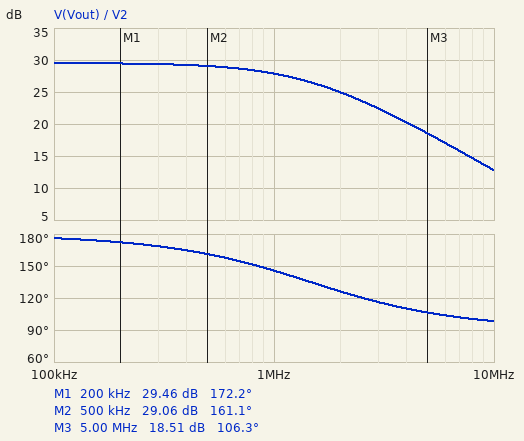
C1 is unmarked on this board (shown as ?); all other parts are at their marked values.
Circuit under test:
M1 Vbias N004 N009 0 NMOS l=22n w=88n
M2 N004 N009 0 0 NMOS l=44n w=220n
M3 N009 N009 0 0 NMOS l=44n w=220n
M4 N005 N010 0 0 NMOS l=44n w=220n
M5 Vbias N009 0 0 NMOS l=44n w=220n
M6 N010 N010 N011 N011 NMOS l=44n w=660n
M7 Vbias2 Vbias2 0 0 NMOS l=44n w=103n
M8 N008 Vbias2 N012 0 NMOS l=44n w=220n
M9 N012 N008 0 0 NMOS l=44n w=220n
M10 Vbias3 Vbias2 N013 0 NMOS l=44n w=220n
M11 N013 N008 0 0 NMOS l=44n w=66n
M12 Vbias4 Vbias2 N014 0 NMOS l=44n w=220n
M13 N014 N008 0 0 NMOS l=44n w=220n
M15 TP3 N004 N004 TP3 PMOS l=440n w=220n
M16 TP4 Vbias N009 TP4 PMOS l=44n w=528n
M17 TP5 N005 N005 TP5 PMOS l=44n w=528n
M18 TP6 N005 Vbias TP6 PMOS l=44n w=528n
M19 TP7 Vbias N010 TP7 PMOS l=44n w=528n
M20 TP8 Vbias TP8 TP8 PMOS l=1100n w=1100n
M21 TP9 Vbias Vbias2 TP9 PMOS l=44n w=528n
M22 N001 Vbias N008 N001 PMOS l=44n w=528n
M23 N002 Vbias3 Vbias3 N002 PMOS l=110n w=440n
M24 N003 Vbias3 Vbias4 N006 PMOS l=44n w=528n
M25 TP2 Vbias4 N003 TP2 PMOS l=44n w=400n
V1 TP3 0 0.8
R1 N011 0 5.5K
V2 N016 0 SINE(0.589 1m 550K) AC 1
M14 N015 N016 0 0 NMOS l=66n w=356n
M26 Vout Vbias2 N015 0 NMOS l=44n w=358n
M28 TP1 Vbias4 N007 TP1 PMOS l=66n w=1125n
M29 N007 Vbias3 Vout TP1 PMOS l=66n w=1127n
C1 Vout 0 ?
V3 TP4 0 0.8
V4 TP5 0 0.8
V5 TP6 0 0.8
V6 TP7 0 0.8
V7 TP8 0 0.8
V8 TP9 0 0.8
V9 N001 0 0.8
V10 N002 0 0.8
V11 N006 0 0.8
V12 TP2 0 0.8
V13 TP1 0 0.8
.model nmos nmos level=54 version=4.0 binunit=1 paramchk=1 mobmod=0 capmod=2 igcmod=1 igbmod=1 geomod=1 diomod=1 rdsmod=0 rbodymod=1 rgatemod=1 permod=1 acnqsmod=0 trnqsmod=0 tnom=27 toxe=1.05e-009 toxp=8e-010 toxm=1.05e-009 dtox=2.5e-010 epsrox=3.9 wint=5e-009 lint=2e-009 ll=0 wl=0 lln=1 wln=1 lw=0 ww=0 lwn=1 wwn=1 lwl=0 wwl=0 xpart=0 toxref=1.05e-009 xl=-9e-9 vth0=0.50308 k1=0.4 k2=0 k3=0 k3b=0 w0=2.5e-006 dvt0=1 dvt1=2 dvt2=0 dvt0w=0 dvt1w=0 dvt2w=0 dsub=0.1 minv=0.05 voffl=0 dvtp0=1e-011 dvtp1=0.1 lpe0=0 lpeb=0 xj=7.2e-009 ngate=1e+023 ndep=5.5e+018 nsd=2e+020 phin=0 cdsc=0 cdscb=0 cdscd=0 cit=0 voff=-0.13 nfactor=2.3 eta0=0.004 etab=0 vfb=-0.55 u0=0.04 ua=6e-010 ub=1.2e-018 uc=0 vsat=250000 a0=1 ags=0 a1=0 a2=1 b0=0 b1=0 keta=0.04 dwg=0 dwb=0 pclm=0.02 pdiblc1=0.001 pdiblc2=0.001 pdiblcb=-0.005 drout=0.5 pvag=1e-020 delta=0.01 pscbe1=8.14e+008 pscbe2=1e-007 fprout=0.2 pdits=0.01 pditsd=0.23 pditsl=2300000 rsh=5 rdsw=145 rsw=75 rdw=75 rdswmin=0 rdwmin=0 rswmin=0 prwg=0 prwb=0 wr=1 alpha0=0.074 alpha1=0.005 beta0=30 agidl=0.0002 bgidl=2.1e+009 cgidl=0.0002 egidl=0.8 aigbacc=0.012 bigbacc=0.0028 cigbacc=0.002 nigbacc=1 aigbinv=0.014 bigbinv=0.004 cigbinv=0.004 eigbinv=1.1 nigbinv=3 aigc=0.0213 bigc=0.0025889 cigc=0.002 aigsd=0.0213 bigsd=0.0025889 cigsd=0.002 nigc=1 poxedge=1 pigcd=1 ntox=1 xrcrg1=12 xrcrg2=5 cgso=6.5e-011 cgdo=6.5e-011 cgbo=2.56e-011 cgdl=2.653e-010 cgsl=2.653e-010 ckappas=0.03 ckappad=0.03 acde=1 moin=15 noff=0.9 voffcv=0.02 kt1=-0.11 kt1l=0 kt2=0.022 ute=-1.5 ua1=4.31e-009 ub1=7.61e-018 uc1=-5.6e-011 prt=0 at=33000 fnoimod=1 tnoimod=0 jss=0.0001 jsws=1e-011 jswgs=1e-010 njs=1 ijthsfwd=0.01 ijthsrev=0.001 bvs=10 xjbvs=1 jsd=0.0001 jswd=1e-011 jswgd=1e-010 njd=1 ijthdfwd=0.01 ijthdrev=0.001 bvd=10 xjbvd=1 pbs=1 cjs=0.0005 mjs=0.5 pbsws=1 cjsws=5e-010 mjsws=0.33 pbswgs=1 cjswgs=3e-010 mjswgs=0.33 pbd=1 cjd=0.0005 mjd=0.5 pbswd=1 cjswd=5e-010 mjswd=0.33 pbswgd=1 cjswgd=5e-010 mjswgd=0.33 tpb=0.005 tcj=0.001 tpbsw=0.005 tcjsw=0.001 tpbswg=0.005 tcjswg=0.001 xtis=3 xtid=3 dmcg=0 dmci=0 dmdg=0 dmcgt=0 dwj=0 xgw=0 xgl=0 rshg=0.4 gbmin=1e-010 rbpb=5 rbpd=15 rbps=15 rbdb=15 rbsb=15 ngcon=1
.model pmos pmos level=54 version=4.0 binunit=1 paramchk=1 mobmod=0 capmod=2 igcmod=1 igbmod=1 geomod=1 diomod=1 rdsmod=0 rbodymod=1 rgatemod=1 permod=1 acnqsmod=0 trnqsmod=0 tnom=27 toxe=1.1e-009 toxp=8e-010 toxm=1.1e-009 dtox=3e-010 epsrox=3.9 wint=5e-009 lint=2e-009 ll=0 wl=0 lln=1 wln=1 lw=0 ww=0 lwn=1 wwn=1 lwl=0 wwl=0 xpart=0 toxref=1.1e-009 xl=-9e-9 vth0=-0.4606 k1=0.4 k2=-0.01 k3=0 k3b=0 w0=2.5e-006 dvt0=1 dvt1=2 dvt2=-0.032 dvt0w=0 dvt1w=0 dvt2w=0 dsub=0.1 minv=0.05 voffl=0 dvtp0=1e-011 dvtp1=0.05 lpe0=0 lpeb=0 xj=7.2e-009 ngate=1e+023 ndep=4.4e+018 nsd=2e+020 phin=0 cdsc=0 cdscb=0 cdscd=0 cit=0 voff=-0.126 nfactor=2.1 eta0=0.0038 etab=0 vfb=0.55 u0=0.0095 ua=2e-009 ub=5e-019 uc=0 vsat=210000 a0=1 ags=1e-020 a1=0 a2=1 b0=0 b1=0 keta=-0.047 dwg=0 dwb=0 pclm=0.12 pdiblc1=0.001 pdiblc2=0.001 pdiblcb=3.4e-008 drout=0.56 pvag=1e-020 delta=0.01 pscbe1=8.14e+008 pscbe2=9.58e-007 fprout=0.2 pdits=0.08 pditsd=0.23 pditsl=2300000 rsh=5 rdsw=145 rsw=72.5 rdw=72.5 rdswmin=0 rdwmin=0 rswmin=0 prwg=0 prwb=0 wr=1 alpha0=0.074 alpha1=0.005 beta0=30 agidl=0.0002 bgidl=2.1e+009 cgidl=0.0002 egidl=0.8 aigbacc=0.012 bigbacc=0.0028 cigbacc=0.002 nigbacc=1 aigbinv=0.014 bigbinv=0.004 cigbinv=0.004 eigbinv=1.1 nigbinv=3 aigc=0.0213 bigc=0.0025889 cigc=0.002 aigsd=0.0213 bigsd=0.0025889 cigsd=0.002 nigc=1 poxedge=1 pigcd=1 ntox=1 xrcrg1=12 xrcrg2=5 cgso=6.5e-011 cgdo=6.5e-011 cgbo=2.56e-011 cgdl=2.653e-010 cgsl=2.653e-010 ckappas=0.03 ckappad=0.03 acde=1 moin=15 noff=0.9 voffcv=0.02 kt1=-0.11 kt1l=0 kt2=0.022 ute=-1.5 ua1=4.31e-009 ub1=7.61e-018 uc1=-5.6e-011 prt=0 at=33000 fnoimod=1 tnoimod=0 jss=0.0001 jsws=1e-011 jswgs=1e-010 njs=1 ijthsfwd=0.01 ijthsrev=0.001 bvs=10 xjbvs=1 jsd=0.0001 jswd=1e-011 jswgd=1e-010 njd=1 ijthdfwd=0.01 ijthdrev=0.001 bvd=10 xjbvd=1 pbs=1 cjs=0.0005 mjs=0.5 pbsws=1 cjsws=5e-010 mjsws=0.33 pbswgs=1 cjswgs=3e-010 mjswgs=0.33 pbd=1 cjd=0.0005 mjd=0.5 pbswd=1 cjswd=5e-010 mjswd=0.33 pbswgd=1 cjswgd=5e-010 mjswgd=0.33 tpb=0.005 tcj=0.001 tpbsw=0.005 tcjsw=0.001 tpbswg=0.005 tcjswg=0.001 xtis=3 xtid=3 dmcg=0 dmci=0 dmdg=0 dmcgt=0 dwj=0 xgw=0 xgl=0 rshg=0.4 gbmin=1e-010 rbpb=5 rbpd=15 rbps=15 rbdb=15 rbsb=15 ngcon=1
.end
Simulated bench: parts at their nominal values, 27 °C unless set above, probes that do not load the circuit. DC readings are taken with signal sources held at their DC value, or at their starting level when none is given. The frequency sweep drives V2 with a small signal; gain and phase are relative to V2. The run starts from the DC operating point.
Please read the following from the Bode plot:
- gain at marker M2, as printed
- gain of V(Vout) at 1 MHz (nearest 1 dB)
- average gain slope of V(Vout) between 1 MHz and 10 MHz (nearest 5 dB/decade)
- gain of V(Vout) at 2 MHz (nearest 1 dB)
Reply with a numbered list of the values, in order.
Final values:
1. 29.06 dB
2. 28 dB
3. -15 dB/decade
4. 25 dB
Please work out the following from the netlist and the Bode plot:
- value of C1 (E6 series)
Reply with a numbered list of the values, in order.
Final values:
1. 330 fF
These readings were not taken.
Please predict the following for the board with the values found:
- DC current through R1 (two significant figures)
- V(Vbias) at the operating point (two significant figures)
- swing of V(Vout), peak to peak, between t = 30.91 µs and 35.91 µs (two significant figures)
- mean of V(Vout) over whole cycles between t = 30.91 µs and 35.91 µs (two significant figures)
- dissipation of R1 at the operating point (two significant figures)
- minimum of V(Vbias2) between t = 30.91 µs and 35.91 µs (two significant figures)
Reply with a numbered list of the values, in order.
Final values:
1. 12 µA
2. 230 mV
3. 56 mV
4. 460 mV
5. 830 nW
6. 620 mV
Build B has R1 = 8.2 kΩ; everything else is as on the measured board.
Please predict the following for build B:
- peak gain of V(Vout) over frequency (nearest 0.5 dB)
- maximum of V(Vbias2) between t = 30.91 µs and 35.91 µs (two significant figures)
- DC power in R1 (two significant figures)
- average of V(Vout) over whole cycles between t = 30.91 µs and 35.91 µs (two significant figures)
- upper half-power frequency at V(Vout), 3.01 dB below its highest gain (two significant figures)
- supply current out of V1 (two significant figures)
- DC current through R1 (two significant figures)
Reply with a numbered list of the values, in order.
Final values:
1. 5.5 dB
2. 580 mV
3. 460 nW
4. 110 mV
5. 12 MHz
6. 2.0 µA
7. 7.5 µA
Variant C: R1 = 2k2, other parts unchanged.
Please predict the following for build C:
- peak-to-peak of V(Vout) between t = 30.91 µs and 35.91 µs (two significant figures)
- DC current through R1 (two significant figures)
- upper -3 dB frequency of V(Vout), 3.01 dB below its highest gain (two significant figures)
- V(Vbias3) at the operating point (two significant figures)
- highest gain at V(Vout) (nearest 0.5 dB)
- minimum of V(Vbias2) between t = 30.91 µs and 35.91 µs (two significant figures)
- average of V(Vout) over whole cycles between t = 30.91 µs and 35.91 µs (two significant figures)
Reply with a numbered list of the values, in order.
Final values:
1. 5.4 mV
2. 32 µA
3. 30 MHz
4. 140 mV
5. 8.5 dB
6. 700 mV
7. 670 mV
